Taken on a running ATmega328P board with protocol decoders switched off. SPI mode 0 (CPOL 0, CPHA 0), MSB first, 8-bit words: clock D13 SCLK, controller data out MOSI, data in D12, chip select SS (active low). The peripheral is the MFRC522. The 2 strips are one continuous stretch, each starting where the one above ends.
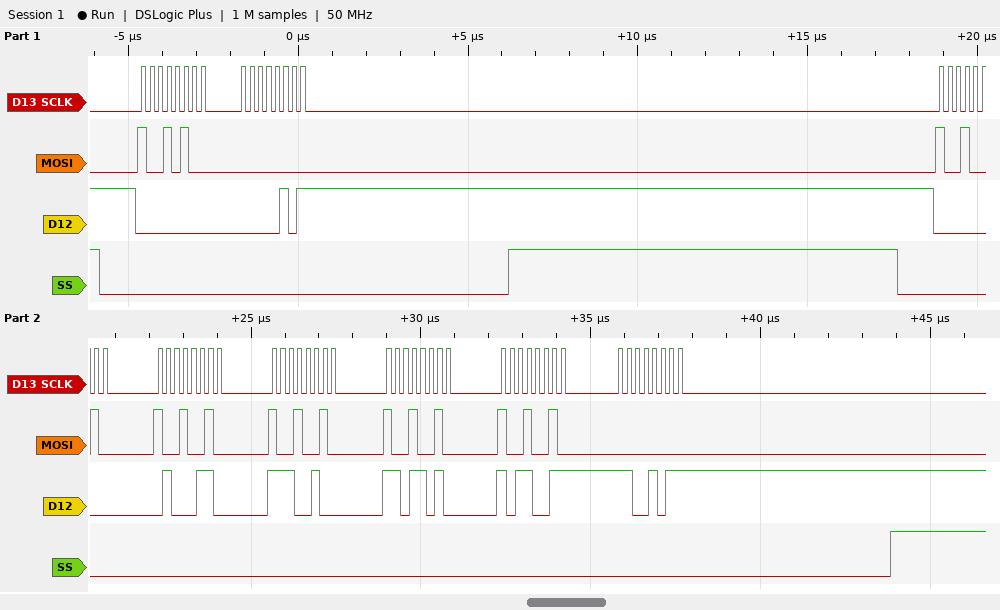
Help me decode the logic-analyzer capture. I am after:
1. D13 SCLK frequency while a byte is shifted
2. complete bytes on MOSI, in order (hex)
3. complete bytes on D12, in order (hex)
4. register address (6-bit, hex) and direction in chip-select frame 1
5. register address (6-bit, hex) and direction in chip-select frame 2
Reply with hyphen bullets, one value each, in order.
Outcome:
- 4 MHz
- 94 00 92 92 92 92 92 00
- 00 05 00 46 E4 DA B3 CB
- 0x0A read
- 0x09 read
